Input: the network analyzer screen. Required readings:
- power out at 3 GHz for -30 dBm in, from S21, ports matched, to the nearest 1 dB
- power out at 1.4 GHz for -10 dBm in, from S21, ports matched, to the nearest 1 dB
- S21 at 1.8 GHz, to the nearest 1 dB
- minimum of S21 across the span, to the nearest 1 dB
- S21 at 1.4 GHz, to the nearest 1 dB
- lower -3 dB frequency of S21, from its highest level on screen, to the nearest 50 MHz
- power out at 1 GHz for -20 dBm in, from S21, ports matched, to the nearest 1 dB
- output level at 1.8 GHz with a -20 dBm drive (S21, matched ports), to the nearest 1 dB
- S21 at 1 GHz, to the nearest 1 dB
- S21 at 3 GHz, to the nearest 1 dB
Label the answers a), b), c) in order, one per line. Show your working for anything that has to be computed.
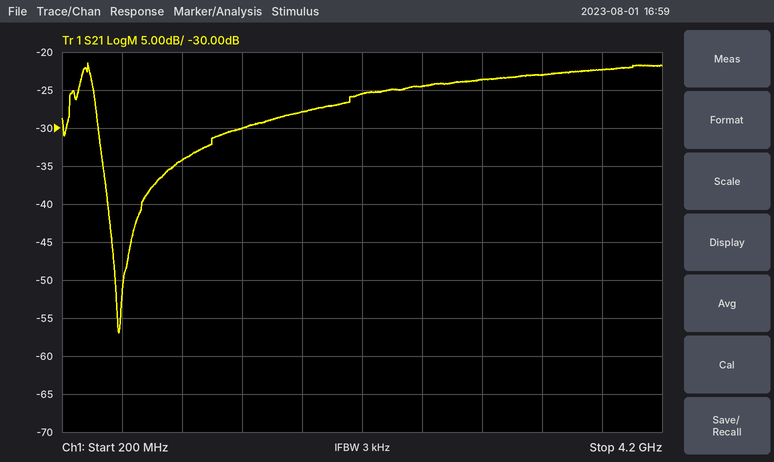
a) -30 dBm + (-24 dB) = -54 dBm
b) -10 dBm + (-30 dB) = -40 dBm
c) -28 dB
d) -57 dB
e) -30 dB
f) 300 MHz
g) -20 dBm + (-34 dB) = -54 dBm
h) -20 dBm + (-28 dB) = -48 dBm
i) -34 dB
j) -24 dB
